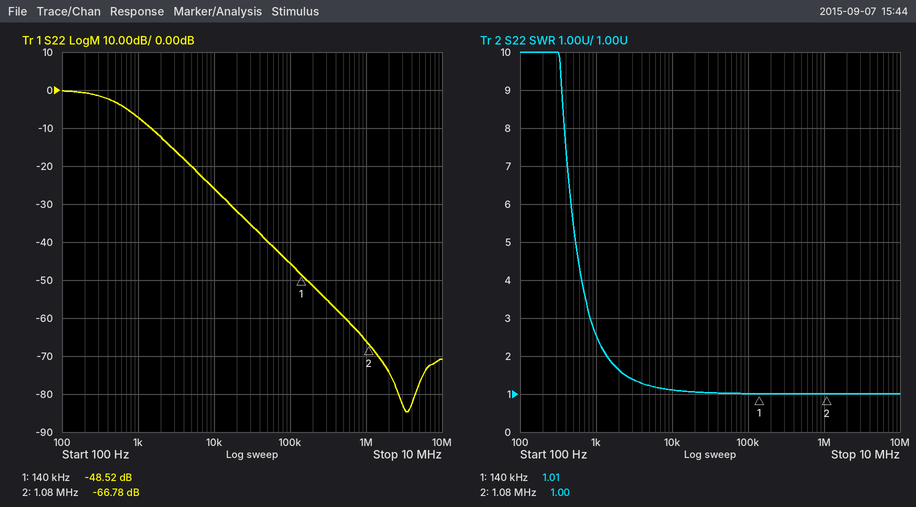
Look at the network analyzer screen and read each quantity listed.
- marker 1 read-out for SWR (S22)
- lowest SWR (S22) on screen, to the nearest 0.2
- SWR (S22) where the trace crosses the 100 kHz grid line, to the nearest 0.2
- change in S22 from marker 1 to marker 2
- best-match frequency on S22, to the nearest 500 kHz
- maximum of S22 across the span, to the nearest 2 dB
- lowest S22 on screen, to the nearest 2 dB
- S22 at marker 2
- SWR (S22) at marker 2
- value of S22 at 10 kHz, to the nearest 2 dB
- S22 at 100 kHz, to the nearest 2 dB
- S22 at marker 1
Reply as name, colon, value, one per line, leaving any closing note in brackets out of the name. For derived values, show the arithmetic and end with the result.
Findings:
marker 1 read-out for SWR: 1.01
lowest SWR (S22) on screen, to the nearest 0.2: 1.0
SWR (S22) where the trace crosses the 100 kHz grid line, to the nearest 0.2: 1.0
change in S22 from marker 1 to marker 2: -66.78 − (-48.52) = -18.26 dB
best-match frequency on S22, to the nearest 500 kHz: 3.5 MHz
maximum of S22 across the span, to the nearest 2 dB: 0 dB
lowest S22 on screen, to the nearest 2 dB: -84 dB
S22 at marker 2: -66.78 dB
SWR (S22) at marker 2: 1.00
value of S22 at 10 kHz, to the nearest 2 dB: -26 dB
S22 at 100 kHz, to the nearest 2 dB: -46 dB
S22 at marker 1: -48.52 dB
